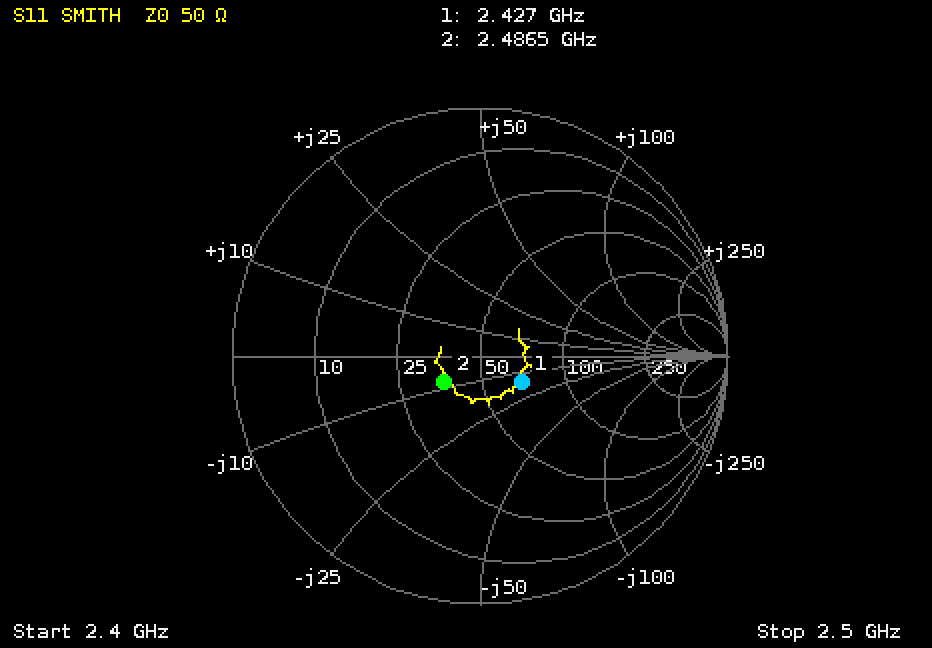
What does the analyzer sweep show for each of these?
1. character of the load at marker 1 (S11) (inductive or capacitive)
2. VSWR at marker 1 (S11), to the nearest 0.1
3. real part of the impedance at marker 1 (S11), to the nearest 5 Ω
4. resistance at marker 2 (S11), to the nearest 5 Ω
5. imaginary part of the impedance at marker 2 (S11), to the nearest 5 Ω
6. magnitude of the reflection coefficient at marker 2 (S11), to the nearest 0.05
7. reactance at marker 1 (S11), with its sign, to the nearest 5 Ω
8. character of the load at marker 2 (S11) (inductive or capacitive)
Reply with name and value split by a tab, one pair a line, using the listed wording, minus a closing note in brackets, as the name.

character of the load at marker 1 (S11)	capacitive
VSWR at marker 1 (S11), to the nearest 0.1	1.5
real part of the impedance at marker 1 (S11), to the nearest 5 Ω	70 Ω
resistance at marker 2 (S11), to the nearest 5 Ω	35 Ω
imaginary part of the impedance at marker 2 (S11), to the nearest 5 Ω	-10 Ω
magnitude of the reflection coefficient at marker 2 (S11), to the nearest 0.05	0.20
reactance at marker 1 (S11), with its sign, to the nearest 5 Ω	-15 Ω
character of the load at marker 2 (S11)	capacitive
